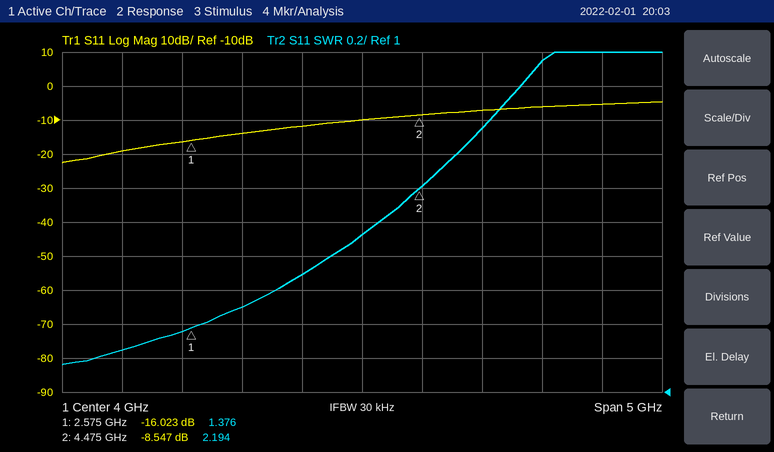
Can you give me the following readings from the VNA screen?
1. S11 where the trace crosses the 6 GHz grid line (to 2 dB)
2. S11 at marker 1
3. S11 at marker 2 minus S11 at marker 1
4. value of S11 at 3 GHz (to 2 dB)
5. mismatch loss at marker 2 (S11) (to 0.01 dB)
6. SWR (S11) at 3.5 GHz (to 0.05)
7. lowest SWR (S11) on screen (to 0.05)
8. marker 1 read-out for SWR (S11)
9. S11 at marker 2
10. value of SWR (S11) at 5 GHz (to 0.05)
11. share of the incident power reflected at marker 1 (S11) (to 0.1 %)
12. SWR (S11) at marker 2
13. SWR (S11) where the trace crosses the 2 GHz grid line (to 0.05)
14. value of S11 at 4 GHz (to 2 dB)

-6 dB
-16.023 dB
7.476 dB
-14 dB
0.65 dB
1.70
1.15
1.376
-8.547 dB
2.55
2.5 %
2.194
1.25
-10 dB
